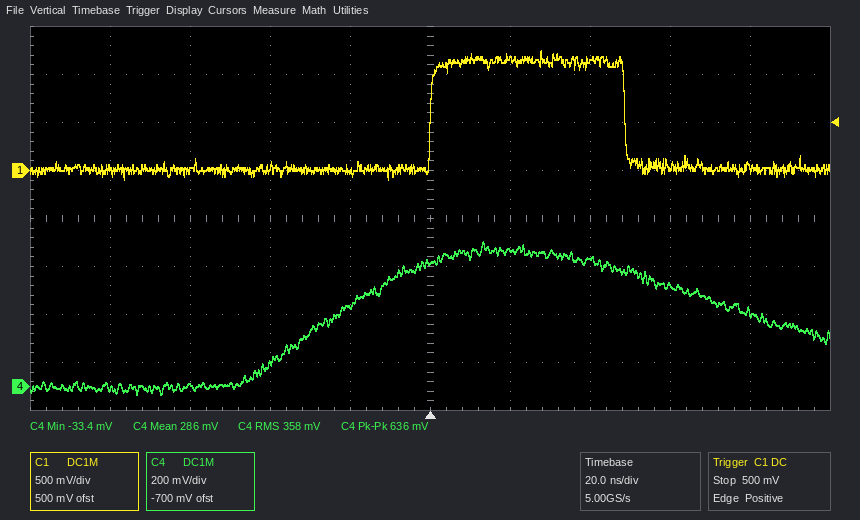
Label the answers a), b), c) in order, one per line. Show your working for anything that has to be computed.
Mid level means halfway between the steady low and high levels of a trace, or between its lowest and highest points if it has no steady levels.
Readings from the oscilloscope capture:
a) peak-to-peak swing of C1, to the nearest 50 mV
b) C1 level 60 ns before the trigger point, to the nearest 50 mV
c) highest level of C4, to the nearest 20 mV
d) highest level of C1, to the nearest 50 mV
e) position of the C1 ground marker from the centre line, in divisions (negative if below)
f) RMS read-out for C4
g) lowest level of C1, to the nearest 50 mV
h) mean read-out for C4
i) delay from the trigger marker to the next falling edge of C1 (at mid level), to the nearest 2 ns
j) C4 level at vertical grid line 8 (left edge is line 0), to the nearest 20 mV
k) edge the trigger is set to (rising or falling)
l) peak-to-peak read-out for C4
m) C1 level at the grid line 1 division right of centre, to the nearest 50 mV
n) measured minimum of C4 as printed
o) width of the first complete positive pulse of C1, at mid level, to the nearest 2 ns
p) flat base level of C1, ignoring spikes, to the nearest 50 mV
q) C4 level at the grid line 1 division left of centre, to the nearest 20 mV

a) 1.25 V − (-100 mV) = 1.35 V
b) 0 mV
c) 600 mV
d) 1.25 V
e) +1.0 div
f) 358 mV
g) -100 mV
h) 286 mV
i) 48 ns
j) 420 mV
k) rising
l) 636 mV
m) 1.15 V
n) -33.4 mV
o) 48 ns
p) 0 mV
q) 340 mV
